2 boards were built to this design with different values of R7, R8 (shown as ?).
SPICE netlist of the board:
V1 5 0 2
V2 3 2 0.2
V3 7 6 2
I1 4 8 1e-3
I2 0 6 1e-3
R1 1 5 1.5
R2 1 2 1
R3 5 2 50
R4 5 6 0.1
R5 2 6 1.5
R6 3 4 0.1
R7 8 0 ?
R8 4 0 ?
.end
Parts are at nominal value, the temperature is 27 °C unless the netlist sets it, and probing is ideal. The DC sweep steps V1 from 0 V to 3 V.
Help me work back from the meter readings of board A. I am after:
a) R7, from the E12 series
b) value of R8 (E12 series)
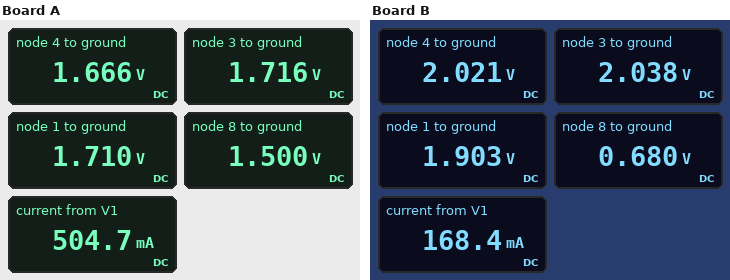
1.5 kΩ
3.3 Ω
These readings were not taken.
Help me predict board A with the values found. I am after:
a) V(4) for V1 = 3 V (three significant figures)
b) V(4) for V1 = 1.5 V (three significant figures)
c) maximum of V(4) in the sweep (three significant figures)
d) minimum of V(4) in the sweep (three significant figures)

2.42 V
1.29 V
2.42 V
151 mV
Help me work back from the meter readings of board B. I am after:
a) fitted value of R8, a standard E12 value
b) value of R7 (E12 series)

12 Ω
680 Ω
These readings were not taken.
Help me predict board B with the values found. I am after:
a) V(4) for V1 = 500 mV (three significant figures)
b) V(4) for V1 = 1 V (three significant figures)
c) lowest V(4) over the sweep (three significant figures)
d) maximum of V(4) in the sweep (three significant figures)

642 mV
1.10 V
183 mV
2.94 V
